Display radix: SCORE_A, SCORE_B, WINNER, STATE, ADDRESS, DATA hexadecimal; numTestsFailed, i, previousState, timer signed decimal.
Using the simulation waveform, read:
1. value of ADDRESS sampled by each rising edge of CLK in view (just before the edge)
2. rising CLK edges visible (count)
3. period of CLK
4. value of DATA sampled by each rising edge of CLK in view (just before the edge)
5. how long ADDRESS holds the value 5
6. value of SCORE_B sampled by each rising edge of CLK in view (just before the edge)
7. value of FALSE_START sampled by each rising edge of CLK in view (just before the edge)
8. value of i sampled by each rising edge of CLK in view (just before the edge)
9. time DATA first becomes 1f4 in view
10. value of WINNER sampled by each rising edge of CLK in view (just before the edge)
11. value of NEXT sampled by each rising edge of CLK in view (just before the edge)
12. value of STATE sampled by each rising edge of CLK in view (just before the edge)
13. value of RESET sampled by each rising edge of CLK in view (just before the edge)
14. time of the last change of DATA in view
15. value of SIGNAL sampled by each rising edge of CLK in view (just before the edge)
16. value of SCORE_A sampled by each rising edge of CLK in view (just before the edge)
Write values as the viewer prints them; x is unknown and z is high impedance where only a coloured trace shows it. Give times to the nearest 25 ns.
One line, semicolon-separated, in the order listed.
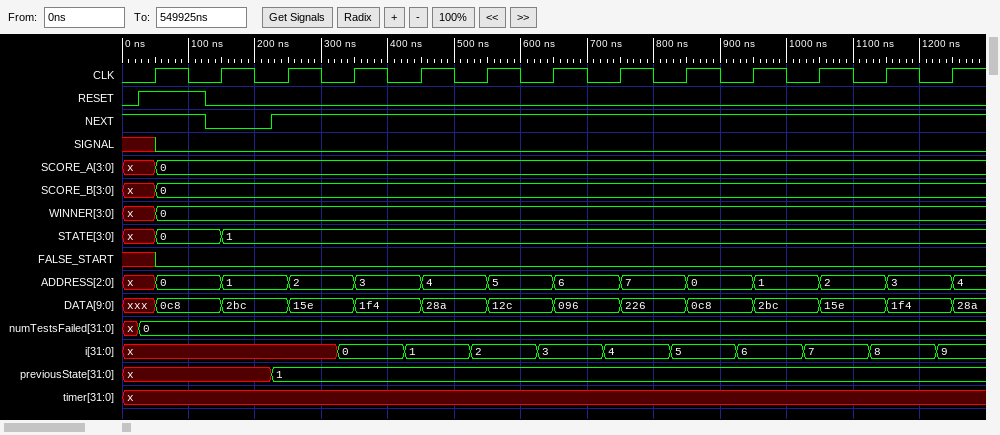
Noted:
x, 0, 1, 2, 3, 4, 5, 6, 7, 0, 1, 2, 3; 13; 100 ns; xxx, 0c8, 2bc, 15e, 1f4, 28a, 12c, 096, 226, 0c8, 2bc, 15e, 1f4; 100 ns; x, 0, 0, 0, 0, 0, 0, 0, 0, 0, 0, 0, 0; x 0 0 0 0 0 0 0 0 0 0 0 0; x, x, x, 0, 1, 2, 3, 4, 5, 6, 7, 8, 9; 350 ns; x, 0, 0, 0, 0, 0, 0, 0, 0, 0, 0, 0, 0; 1 0 1 1 1 1 1 1 1 1 1 1 1; x, 0, 1, 1, 1, 1, 1, 1, 1, 1, 1, 1, 1; 1 0 0 0 0 0 0 0 0 0 0 0 0; 1250 ns; x 0 0 0 0 0 0 0 0 0 0 0 0; x, 0, 0, 0, 0, 0, 0, 0, 0, 0, 0, 0, 0
